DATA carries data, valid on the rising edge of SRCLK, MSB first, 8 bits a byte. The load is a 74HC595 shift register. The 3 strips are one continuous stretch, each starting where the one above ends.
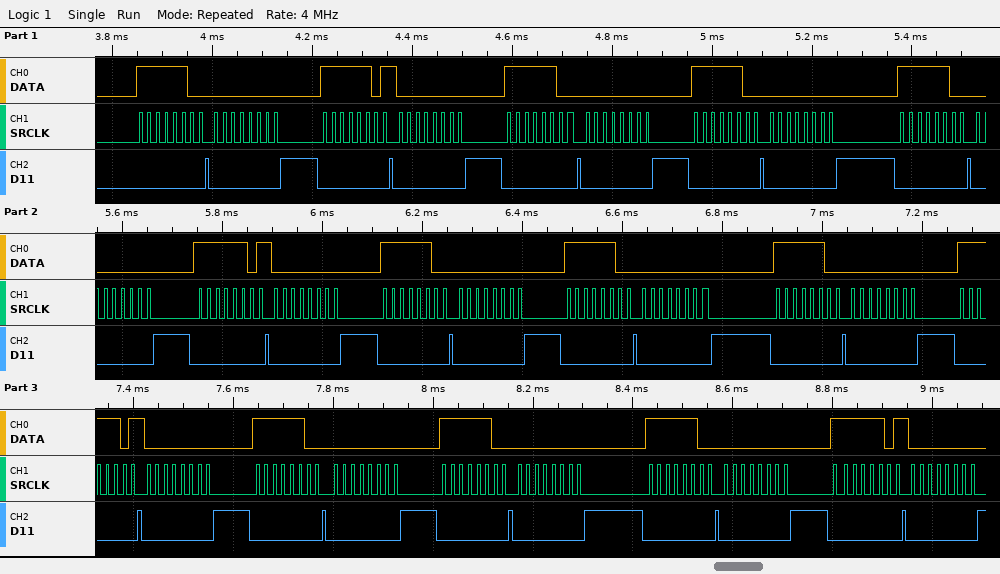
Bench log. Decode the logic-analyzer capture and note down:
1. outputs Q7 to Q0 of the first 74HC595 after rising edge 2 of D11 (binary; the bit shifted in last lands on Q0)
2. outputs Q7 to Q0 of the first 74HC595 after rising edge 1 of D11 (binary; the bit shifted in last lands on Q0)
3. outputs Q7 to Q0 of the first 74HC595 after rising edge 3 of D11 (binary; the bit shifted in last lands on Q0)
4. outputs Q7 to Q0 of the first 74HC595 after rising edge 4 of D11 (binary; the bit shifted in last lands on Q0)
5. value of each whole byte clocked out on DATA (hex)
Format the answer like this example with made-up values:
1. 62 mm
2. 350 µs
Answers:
1. 00000000
2. 11111100
3. 11111101
4. 00000000
5. FC 00 FD 00 FC 00 FC 00 FC 00 FD 00 FC 00 FC 00 FC 00 FD 00 FC 00 FC 00 FC 00 FD 00
